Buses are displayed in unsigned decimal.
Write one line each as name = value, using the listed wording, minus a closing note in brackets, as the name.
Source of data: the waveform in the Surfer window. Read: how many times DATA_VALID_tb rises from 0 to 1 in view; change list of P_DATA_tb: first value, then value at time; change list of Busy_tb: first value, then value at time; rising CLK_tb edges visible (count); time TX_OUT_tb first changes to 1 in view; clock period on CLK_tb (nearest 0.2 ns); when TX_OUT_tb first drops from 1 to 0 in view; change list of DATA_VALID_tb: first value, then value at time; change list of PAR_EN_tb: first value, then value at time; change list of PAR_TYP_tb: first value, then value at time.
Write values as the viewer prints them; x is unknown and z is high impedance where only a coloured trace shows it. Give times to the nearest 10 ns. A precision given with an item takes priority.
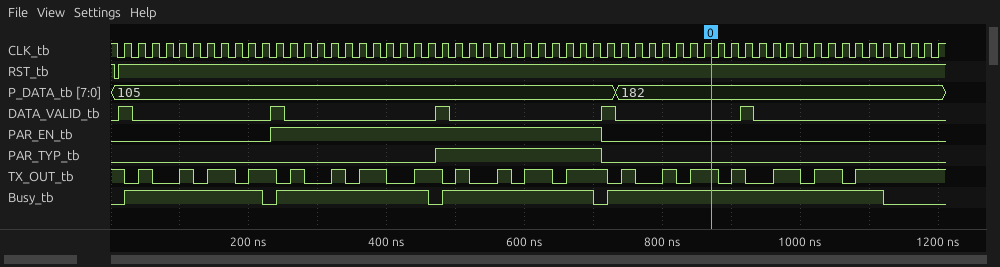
how many times DATA_VALID_tb rises from 0 to 1 in view = 5
change list of P_DATA_tb: first value, then value at time = 105, 182 at 730 ns
change list of Busy_tb: first value, then value at time = 0, 1 at 20 ns, 0 at 220 ns, 1 at 240 ns, 0 at 460 ns, 1 at 480 ns, 0 at 700 ns, 1 at 720 ns, 0 at 1120 ns
rising CLK_tb edges visible = 60
time TX_OUT_tb first changes to 1 in view = 40 ns
clock period on CLK_tb = 20 ns
when TX_OUT_tb first drops from 1 to 0 in view = 20 ns
change list of DATA_VALID_tb: first value, then value at time = 0, 1 at 10 ns, 0 at 30 ns, 1 at 230 ns, 0 at 250 ns, 1 at 470 ns, 0 at 490 ns, 1 at 710 ns, 0 at 730 ns, 1 at 910 ns, 0 at 930 ns
change list of PAR_EN_tb: first value, then value at time = 0, 1 at 230 ns, 0 at 710 ns
change list of PAR_TYP_tb: first value, then value at time = 0, 1 at 470 ns, 0 at 710 ns
